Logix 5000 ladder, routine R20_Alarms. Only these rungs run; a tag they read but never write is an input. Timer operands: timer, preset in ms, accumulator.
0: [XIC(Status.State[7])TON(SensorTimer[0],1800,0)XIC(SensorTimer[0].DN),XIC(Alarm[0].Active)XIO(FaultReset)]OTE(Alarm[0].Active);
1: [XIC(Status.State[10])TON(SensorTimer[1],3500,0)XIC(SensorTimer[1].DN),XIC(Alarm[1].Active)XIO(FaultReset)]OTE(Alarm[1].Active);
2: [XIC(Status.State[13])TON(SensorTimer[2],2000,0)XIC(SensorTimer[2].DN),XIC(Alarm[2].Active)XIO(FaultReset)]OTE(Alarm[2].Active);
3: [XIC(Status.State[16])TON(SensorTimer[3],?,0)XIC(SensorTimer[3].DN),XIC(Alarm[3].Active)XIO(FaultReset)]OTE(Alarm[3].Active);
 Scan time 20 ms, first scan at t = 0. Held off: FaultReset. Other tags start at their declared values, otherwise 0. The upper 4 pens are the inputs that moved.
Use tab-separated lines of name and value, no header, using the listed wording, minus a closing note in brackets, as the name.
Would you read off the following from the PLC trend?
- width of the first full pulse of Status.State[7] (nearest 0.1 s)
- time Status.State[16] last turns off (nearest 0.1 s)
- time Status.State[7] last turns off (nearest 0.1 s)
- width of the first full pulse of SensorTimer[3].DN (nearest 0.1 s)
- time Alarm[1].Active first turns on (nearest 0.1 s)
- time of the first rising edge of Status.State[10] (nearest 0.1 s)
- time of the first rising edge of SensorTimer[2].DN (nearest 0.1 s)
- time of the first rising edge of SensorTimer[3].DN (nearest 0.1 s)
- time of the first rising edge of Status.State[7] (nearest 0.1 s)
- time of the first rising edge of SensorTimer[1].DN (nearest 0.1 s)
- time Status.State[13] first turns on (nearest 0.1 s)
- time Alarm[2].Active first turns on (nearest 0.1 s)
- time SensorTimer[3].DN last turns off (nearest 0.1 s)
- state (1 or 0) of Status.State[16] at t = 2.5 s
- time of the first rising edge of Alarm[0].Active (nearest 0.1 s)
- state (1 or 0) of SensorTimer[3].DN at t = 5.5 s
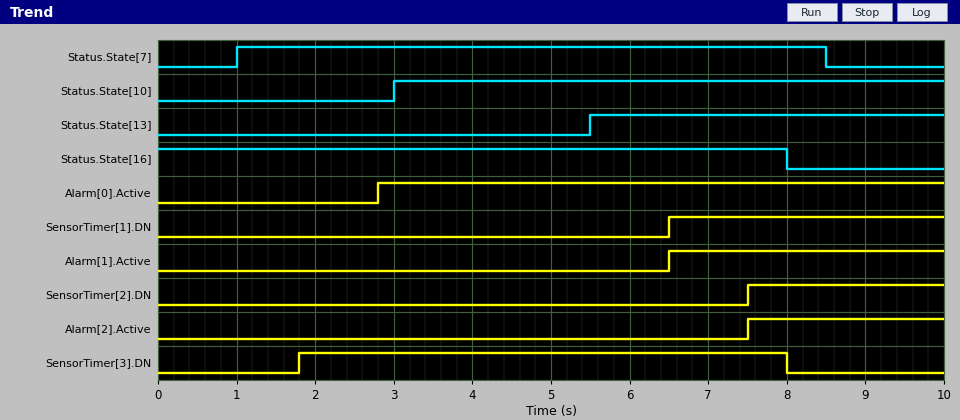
width of the first full pulse of Status.State[7]	7.5 s
time Status.State[16] last turns off	8.0 s
time Status.State[7] last turns off	8.5 s
width of the first full pulse of SensorTimer[3].DN	6.2 s
time Alarm[1].Active first turns on	6.5 s
time of the first rising edge of Status.State[10]	3.0 s
time of the first rising edge of SensorTimer[2].DN	7.5 s
time of the first rising edge of SensorTimer[3].DN	1.8 s
time of the first rising edge of Status.State[7]	1.0 s
time of the first rising edge of SensorTimer[1].DN	6.5 s
time Status.State[13] first turns on	5.5 s
time Alarm[2].Active first turns on	7.5 s
time SensorTimer[3].DN last turns off	8.0 s
state (1 or 0) of Status.State[16] at t = 2.5 s	1
time of the first rising edge of Alarm[0].Active	2.8 s
state (1 or 0) of SensorTimer[3].DN at t = 5.5 s	1
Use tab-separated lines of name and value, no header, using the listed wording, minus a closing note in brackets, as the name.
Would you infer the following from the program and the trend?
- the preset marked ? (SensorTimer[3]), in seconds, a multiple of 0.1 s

the preset marked ? (SensorTimer[3]), in seconds, a multiple of 0.1 s	1.8 s
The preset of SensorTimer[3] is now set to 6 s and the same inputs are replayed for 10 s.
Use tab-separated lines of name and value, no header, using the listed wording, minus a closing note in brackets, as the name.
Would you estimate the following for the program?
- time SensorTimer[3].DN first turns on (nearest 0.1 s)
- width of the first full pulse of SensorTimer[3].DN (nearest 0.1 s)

time SensorTimer[3].DN first turns on	6.0 s
width of the first full pulse of SensorTimer[3].DN	2.0 s
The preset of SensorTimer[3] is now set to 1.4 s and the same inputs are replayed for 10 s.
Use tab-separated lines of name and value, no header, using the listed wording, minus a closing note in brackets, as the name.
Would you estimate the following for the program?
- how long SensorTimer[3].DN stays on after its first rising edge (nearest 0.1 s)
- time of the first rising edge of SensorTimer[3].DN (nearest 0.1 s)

how long SensorTimer[3].DN stays on after its first rising edge	6.6 s
time of the first rising edge of SensorTimer[3].DN	1.4 s
